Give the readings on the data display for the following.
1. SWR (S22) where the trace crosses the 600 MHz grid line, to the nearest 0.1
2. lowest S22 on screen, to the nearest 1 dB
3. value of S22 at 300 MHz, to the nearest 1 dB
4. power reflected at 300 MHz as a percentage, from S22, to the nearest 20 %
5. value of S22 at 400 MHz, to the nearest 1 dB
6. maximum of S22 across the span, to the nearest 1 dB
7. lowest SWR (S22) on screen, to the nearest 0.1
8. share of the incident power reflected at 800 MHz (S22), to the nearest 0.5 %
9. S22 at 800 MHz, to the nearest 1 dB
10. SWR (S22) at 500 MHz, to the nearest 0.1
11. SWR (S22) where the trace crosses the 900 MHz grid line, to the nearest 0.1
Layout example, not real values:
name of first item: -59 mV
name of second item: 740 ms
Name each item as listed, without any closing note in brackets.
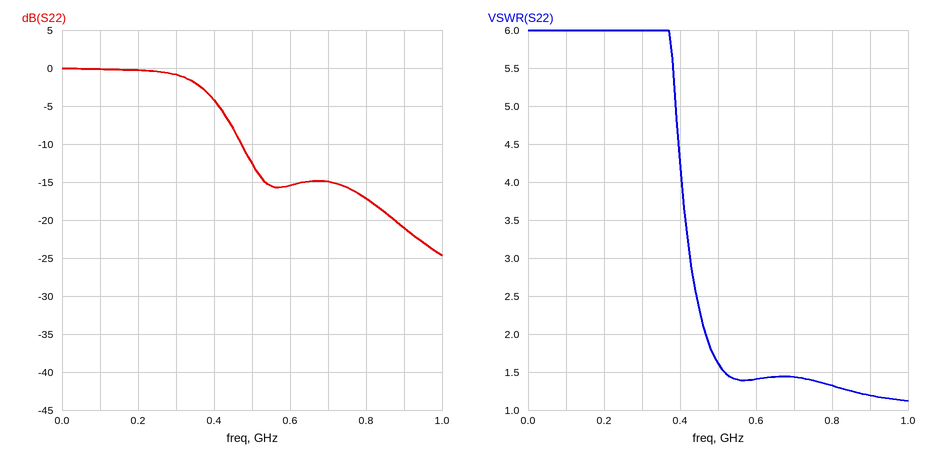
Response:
SWR (S22) where the trace crosses the 600 MHz grid line, to the nearest 0.1: 1.4
lowest S22 on screen, to the nearest 1 dB: -25 dB
value of S22 at 300 MHz, to the nearest 1 dB: -1 dB
power reflected at 300 MHz as a percentage, from S22, to the nearest 20 %: 80 %
value of S22 at 400 MHz, to the nearest 1 dB: -4 dB
maximum of S22 across the span, to the nearest 1 dB: 0 dB
lowest SWR (S22) on screen, to the nearest 0.1: 1.1
share of the incident power reflected at 800 MHz (S22), to the nearest 0.5 %: 2.0 %
S22 at 800 MHz, to the nearest 1 dB: -17 dB
SWR (S22) at 500 MHz, to the nearest 0.1: 1.6
SWR (S22) where the trace crosses the 900 MHz grid line, to the nearest 0.1: 1.2
